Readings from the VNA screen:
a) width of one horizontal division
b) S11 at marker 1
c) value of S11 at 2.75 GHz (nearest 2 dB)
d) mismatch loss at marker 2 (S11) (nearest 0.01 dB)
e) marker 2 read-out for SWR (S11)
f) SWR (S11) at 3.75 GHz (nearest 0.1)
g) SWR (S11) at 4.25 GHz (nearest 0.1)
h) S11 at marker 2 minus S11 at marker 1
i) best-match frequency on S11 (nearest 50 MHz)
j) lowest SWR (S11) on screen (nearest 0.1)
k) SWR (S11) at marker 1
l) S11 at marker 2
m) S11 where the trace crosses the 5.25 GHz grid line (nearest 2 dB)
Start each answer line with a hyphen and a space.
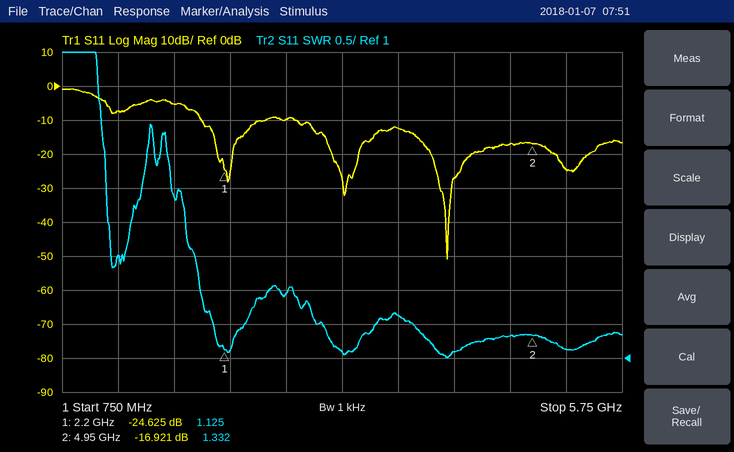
- 500 MHz
- -24.625 dB
- -10 dB
- 0.09 dB
- 1.332
- 1.6
- 1.1
- 7.704 dB
- 4.20 GHz
- 1.0
- 1.125
- -16.921 dB
- -24 dB
